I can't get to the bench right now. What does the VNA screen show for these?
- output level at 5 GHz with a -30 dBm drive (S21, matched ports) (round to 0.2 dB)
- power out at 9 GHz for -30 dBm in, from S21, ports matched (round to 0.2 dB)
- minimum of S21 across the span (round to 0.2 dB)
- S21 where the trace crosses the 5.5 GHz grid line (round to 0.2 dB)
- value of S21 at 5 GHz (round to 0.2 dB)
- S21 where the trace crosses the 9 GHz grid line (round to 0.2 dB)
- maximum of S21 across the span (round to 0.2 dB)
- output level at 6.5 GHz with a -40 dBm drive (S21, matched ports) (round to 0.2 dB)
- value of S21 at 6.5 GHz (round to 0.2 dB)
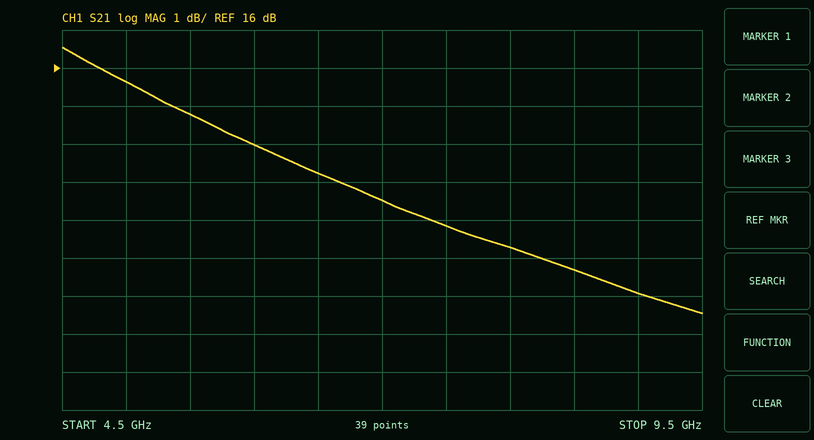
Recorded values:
-14.4 dBm
-20.0 dBm
9.6 dB
14.8 dB
15.6 dB
10.0 dB
16.6 dB
-26.8 dBm
13.2 dB
